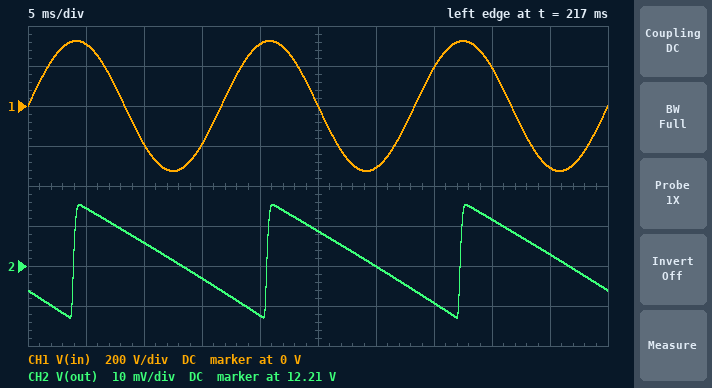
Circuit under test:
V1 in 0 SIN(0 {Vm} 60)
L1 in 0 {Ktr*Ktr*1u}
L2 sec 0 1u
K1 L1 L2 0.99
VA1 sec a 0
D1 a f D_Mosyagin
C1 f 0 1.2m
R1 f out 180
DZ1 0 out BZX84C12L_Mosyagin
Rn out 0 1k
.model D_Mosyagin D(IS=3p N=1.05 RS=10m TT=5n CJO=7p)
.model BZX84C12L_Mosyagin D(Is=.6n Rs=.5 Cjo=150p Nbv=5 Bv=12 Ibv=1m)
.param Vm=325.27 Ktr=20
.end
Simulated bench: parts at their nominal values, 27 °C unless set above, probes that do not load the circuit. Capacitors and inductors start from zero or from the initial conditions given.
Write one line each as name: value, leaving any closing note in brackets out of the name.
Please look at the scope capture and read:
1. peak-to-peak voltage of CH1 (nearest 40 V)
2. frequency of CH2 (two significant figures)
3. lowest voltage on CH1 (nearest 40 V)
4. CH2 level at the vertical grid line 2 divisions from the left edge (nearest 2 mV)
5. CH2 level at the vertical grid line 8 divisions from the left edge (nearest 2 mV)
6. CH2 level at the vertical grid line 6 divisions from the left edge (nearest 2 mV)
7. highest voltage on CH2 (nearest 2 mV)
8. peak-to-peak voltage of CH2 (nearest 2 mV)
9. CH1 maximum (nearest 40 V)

peak-to-peak voltage of CH1: 640 V
frequency of CH2: 60 Hz
lowest voltage on CH1: -320 V
CH2 level at the vertical grid line 2 divisions from the left edge: 12.216 V
CH2 level at the vertical grid line 8 divisions from the left edge: 12.222 V
CH2 level at the vertical grid line 6 divisions from the left edge: 12.210 V
highest voltage on CH2: 12.226 V
peak-to-peak voltage of CH2: 28 mV
CH1 maximum: 320 V
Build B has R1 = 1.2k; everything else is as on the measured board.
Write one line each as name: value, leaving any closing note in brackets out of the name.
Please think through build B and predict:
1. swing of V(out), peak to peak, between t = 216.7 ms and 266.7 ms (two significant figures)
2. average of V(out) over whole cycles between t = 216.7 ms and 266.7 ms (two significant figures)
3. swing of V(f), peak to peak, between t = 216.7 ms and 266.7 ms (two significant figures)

swing of V(out), peak to peak, between t = 216.7 ms and 266.7 ms: 42 mV
average of V(out) over whole cycles between t = 216.7 ms and 266.7 ms: 7.0 V
swing of V(f), peak to peak, between t = 216.7 ms and 266.7 ms: 93 mV
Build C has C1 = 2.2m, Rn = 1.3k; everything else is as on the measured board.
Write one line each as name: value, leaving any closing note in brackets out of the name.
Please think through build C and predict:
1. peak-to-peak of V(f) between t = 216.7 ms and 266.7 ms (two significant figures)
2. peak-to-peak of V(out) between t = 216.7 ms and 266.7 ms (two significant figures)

peak-to-peak of V(f) between t = 216.7 ms and 266.7 ms: 120 mV
peak-to-peak of V(out) between t = 216.7 ms and 266.7 ms: 11 mV
